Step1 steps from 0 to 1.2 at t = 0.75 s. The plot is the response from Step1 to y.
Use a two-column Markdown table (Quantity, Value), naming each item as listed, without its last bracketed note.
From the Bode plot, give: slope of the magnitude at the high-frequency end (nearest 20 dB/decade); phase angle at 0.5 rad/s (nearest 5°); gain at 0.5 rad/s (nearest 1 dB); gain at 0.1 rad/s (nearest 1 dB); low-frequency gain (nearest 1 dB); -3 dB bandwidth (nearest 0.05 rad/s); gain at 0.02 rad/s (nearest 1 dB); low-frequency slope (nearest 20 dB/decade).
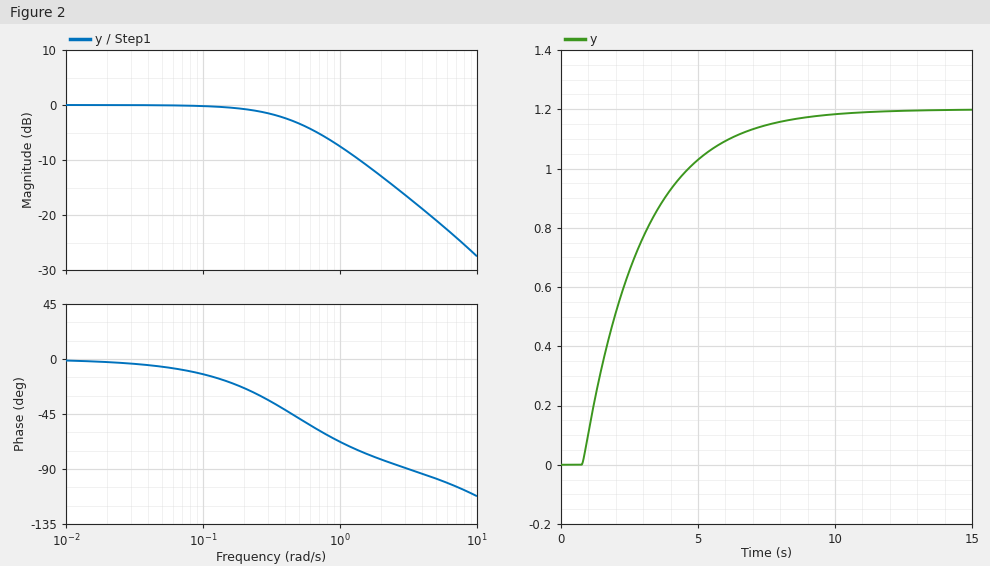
| Quantity | Value |
|---|---|
| slope of the magnitude at the high-frequency end | -20 dB/decade |
| phase angle at 0.5 rad/s | -50° |
| gain at 0.5 rad/s | -3 dB |
| gain at 0.1 rad/s | 0 dB |
| low-frequency gain | 0 dB |
| -3 dB bandwidth | 0.45 rad/s |
| gain at 0.02 rad/s | 0 dB |
| low-frequency slope | 0 dB/decade |
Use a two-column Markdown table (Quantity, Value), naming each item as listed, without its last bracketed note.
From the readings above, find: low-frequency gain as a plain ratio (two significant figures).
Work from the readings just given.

| Quantity | Value |
|---|---|
| low-frequency gain as a plain ratio | 1.0 |
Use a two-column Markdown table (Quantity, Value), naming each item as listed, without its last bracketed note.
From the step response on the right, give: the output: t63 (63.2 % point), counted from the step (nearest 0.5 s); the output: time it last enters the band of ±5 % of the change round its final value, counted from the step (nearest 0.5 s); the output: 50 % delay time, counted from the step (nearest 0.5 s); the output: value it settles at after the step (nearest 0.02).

| Quantity | Value |
|---|---|
| the output: t63 (63.2 % point), counted from the step | 2.0 s |
| the output: time it last enters the band of ±5 % of the change round its final value, counted from the step | 6.5 s |
| the output: 50 % delay time, counted from the step | 1.5 s |
| the output: value it settles at after the step | 1.20 |
